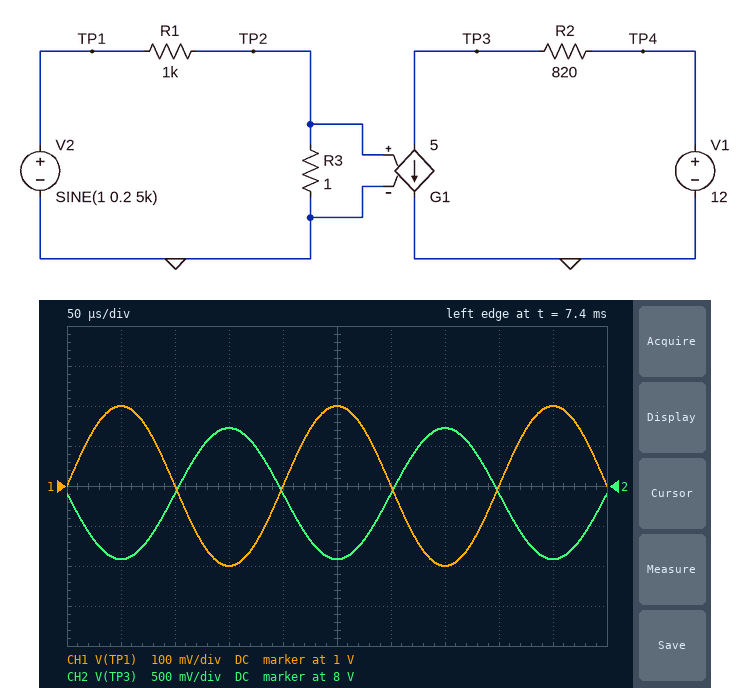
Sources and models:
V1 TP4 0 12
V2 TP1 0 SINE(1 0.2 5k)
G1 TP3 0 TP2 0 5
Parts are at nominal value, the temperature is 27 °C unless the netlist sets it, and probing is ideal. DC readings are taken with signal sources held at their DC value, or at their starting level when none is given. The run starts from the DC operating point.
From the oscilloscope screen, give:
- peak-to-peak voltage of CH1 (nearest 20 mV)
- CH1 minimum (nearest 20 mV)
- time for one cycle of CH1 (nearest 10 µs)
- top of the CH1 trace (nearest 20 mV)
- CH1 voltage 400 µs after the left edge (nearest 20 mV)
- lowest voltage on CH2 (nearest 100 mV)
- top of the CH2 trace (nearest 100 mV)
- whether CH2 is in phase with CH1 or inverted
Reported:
400 mV
800 mV
200 µs
1.20 V
1.00 V
7.1 V
8.7 V
inverted
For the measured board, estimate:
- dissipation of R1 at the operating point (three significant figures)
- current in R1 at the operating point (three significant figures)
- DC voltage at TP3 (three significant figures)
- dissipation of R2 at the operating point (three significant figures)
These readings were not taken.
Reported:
998 µW
999 µA
7.90 V
20.5 mW
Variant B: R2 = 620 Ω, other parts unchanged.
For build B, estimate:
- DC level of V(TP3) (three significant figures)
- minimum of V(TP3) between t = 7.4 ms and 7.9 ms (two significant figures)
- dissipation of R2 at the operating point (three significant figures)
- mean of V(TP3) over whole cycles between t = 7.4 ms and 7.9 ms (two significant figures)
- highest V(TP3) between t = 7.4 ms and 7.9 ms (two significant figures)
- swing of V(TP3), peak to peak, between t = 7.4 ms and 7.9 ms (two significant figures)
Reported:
8.90 V
8.3 V
15.5 mW
8.9 V
9.5 V
1.2 V
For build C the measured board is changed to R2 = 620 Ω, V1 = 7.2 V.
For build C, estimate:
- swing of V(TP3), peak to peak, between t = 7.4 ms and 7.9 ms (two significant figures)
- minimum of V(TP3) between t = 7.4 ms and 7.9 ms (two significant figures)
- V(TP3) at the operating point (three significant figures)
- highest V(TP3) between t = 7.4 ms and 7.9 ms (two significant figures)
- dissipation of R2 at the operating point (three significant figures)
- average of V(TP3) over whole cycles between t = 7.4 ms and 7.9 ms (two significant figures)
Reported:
1.2 V
3.5 V
4.10 V
4.7 V
15.5 mW
4.1 V
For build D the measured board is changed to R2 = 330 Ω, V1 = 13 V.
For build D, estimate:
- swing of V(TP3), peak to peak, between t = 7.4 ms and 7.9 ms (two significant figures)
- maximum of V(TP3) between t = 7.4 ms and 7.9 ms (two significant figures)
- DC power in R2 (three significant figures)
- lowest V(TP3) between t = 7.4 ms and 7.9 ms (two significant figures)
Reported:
660 mV
12 V
8.23 mW
11 V
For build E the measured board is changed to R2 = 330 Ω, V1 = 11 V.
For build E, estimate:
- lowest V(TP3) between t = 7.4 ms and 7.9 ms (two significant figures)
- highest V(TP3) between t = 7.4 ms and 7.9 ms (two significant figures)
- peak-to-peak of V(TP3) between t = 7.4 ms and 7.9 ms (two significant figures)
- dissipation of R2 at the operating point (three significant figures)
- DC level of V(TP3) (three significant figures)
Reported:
9.0 V
9.7 V
660 mV
8.23 mW
9.35 V
